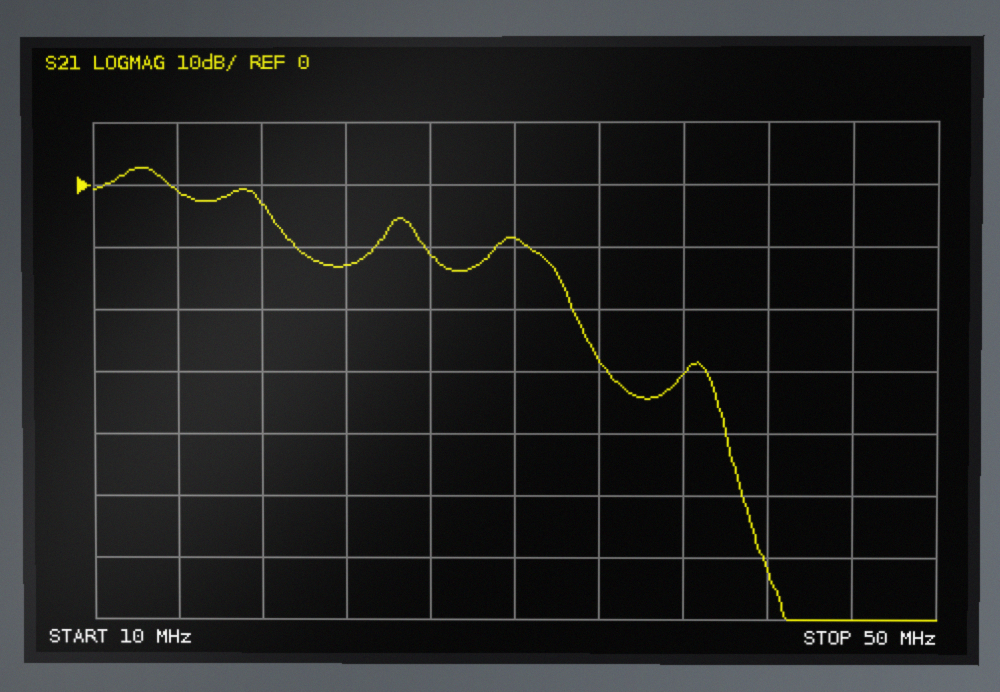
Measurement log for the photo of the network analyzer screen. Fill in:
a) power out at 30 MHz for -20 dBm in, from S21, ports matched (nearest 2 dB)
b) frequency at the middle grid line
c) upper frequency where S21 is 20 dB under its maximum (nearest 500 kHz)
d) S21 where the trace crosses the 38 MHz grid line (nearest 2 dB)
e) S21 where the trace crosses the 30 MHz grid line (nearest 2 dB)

-28 dBm
30 MHz
32.5 MHz
-30 dB
-8 dB
